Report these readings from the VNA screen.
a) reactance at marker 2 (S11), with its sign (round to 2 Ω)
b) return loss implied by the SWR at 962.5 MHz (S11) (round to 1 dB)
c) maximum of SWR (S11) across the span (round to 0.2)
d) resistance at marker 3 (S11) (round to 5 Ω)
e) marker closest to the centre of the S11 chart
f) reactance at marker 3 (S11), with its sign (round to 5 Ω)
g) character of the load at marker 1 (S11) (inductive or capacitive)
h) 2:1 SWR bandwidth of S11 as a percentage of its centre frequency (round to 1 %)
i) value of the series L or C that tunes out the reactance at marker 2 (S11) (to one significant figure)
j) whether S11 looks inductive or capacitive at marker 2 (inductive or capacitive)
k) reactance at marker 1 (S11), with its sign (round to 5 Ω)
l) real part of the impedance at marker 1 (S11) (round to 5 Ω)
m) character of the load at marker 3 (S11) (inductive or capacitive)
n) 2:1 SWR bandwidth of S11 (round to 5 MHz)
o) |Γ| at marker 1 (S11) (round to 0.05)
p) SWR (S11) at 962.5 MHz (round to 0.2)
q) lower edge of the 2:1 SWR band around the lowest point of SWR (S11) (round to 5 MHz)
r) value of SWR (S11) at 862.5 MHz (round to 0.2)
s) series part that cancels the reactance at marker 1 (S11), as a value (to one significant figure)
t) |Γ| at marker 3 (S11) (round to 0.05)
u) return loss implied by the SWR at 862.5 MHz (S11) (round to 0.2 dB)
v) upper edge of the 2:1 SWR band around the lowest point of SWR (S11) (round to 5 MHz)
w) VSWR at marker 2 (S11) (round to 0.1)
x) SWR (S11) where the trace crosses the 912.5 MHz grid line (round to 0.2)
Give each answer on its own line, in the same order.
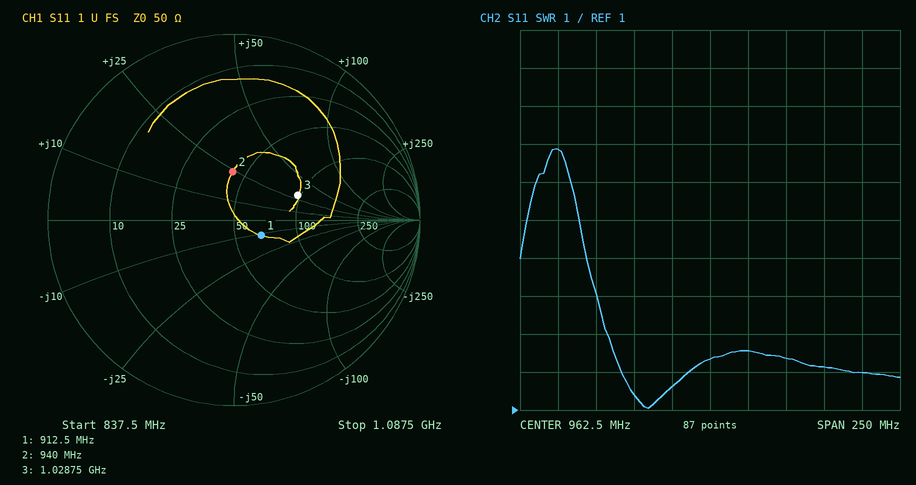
+24 Ω
8 dB
7.8
95 Ω
marker 1
+30 Ω
capacitive
5 %
7 pF
inductive
-10 Ω
65 Ω
inductive
45 MHz
0.15
2.4
905 MHz
7.8
2 nH
0.35
2.2 dB
950 MHz
1.7
1.4
